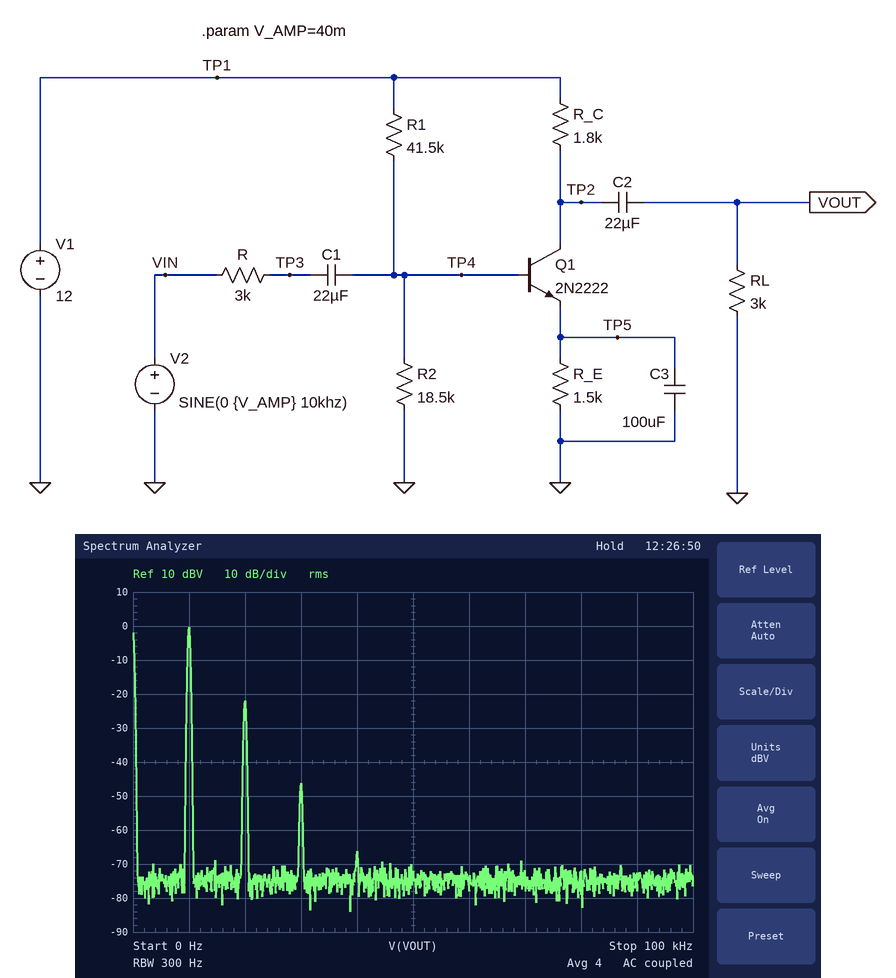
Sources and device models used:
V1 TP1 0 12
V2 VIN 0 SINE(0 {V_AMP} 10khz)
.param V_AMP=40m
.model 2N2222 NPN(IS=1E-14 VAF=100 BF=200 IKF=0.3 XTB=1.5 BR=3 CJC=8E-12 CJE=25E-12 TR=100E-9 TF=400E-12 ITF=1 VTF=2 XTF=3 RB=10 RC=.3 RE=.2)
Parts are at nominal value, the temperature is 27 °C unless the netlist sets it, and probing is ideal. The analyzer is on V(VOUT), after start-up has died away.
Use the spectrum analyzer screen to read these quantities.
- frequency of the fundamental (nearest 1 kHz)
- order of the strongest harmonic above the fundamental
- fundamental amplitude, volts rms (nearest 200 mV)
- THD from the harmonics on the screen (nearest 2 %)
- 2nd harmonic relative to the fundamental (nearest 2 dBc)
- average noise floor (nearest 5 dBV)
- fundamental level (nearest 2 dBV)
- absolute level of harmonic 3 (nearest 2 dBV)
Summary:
10 kHz
2
1.0 V
8 %
-22 dBc
-75 dBV
0 dBV
-46 dBV
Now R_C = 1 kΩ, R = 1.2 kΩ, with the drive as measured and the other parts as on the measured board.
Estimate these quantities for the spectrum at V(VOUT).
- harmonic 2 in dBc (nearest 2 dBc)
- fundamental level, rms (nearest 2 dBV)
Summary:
-16 dBc
0 dBV
